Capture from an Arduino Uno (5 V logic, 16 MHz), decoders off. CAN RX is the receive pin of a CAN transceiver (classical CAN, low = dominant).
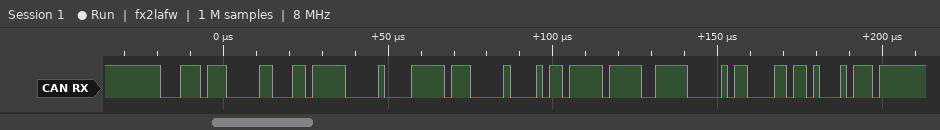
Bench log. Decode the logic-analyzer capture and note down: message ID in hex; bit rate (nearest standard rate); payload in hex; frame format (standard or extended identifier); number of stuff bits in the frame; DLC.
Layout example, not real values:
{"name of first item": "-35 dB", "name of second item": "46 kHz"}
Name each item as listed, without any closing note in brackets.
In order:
{"message ID in hex": "0x1DC", "bit rate": "500 kbit/s", "payload in hex": "DF 00 FF 00 5B FF 7C 18", "frame format": "standard", "number of stuff bits in the frame": "9", "DLC": "8"}
